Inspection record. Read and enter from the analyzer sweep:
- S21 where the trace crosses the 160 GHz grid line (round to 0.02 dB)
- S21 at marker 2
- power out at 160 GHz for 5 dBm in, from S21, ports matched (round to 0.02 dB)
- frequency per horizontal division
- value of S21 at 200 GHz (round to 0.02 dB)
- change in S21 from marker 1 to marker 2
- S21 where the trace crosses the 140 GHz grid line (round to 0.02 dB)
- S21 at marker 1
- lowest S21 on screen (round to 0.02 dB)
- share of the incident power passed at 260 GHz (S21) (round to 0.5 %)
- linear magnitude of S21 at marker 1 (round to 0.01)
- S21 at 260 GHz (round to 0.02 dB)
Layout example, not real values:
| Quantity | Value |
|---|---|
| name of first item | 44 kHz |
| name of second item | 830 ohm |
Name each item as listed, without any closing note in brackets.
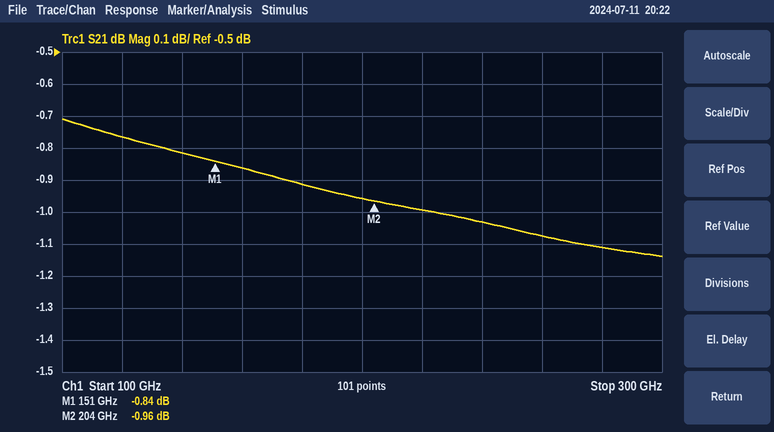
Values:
| Quantity | Value |
|---|---|
| S21 where the trace crosses the 160 GHz grid line | -0.86 dB |
| S21 at marker 2 | -0.96 dB |
| power out at 160 GHz for 5 dBm in, from S21, ports matched | 4.14 dBm |
| frequency per horizontal division | 20 GHz |
| value of S21 at 200 GHz | -0.96 dB |
| change in S21 from marker 1 to marker 2 | -0.12 dB |
| S21 where the trace crosses the 140 GHz grid line | -0.82 dB |
| S21 at marker 1 | -0.84 dB |
| lowest S21 on screen | -1.14 dB |
| share of the incident power passed at 260 GHz (S21) | 78.0 % |
| linear magnitude of S21 at marker 1 | 0.91 |
| S21 at 260 GHz | -1.08 dB |
